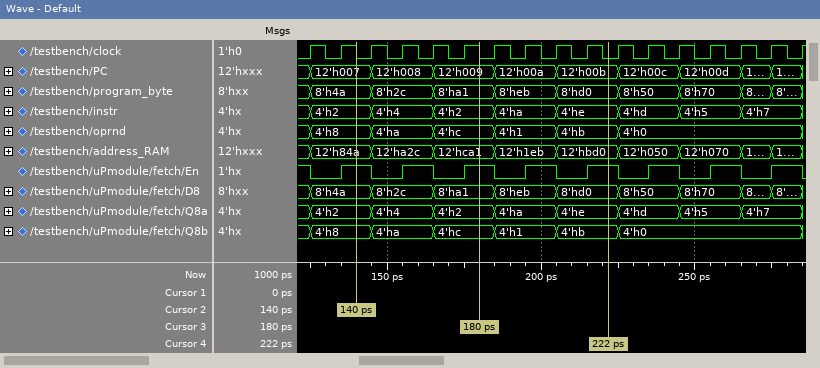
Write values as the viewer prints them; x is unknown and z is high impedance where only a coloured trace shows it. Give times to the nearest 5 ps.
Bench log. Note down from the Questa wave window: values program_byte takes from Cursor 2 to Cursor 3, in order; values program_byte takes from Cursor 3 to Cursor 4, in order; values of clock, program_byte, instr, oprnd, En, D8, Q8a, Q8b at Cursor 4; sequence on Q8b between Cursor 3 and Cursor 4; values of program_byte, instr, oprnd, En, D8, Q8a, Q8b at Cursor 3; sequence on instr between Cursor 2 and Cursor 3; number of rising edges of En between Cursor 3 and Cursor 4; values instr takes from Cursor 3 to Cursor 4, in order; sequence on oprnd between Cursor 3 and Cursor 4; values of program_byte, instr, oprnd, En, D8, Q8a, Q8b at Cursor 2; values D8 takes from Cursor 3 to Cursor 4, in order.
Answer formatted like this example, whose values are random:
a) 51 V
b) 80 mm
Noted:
a) 8'h4a, 8'h2c, 8'ha1
b) 8'ha1, 8'heb, 8'hd0
c) clock=0, program_byte=8'hd0, instr=4'he, oprnd=4'hb, En=1, D8=8'hd0, Q8a=4'he, Q8b=4'hb
d) 4'hc, 4'h1, 4'hb
e) program_byte=8'ha1, instr=4'h2, oprnd=4'hc, En=1, D8=8'ha1, Q8a=4'h2, Q8b=4'hc
f) 4'h2, 4'h4, 4'h2
g) 2
h) 4'h2, 4'ha, 4'he
i) 4'hc, 4'h1, 4'hb
j) program_byte=8'h4a, instr=4'h2, oprnd=4'h8, En=1, D8=8'h4a, Q8a=4'h2, Q8b=4'h8
k) 8'ha1, 8'heb, 8'hd0
